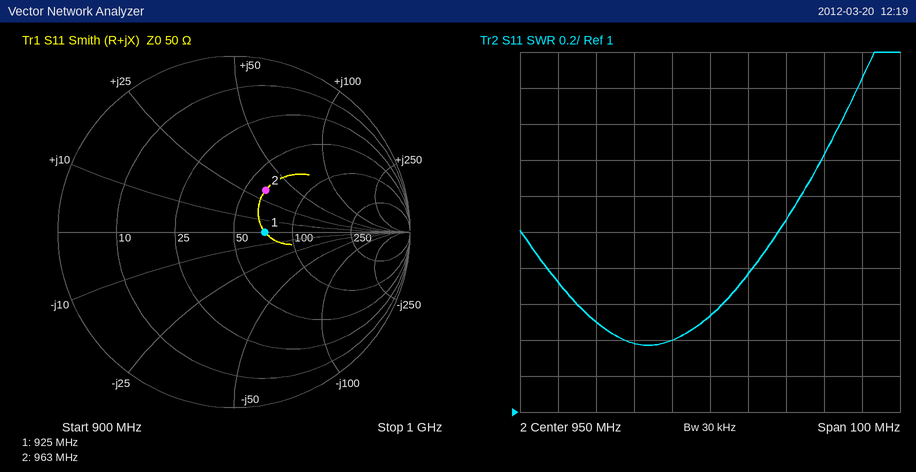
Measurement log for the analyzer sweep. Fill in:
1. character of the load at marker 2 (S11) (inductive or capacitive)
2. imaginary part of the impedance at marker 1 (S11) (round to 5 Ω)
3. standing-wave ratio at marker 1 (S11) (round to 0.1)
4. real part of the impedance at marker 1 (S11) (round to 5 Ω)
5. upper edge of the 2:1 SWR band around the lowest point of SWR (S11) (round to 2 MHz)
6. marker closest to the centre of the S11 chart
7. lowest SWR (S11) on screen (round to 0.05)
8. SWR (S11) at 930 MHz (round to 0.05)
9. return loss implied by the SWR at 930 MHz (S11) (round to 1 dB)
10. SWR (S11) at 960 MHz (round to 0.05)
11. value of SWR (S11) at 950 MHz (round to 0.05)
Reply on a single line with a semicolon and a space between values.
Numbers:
inductive; 0 Ω; 1.4; 70 Ω; 968 MHz; marker 1; 1.35; 1.40; 16 dB; 1.75; 1.55
